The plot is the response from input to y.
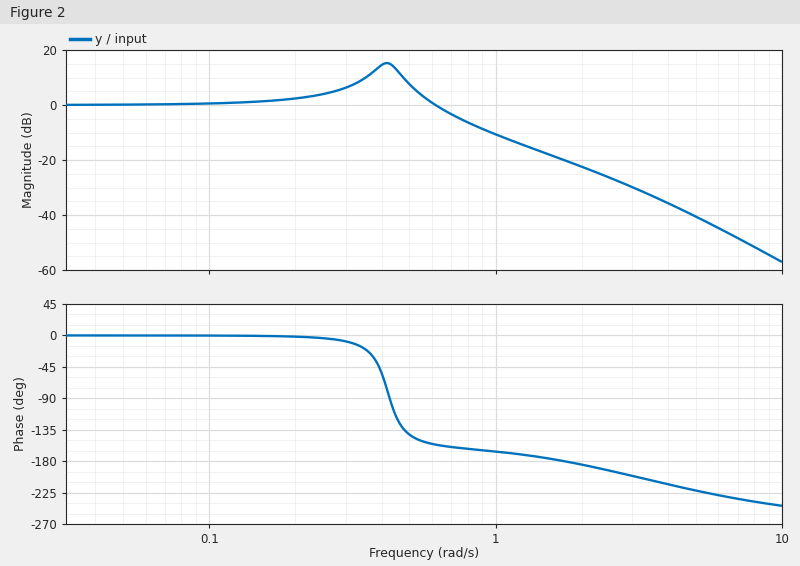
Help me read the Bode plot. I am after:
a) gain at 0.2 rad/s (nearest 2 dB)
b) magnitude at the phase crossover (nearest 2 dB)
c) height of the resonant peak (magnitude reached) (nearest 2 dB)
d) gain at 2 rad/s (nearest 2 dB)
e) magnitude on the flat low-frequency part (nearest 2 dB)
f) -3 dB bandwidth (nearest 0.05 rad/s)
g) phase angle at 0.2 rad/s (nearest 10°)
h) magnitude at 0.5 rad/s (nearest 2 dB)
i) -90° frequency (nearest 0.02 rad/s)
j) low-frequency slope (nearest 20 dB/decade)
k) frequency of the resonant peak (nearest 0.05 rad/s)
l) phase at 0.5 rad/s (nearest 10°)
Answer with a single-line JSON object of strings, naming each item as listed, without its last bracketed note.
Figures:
{"gain at 0.2 rad/s": "2 dB", "magnitude at the phase crossover": "-20 dB", "height of the resonant peak (magnitude reached)": "16 dB", "gain at 2 rad/s": "-22 dB", "magnitude on the flat low-frequency part": "0 dB", "-3 dB bandwidth": "0.70 rad/s", "phase angle at 0.2 rad/s": "0°", "magnitude at 0.5 rad/s": "8 dB", "-90° frequency": "0.42 rad/s", "low-frequency slope": "0 dB/decade", "frequency of the resonant peak": "0.40 rad/s", "phase at 0.5 rad/s": "-140°"}
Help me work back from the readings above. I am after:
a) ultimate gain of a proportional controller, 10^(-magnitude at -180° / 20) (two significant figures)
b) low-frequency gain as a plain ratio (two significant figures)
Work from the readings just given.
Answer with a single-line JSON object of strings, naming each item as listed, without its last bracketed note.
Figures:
{"ultimate gain of a proportional controller, 10^(-magnitude at -180° / 20)": "10", "low-frequency gain as a plain ratio": "1.0"}
